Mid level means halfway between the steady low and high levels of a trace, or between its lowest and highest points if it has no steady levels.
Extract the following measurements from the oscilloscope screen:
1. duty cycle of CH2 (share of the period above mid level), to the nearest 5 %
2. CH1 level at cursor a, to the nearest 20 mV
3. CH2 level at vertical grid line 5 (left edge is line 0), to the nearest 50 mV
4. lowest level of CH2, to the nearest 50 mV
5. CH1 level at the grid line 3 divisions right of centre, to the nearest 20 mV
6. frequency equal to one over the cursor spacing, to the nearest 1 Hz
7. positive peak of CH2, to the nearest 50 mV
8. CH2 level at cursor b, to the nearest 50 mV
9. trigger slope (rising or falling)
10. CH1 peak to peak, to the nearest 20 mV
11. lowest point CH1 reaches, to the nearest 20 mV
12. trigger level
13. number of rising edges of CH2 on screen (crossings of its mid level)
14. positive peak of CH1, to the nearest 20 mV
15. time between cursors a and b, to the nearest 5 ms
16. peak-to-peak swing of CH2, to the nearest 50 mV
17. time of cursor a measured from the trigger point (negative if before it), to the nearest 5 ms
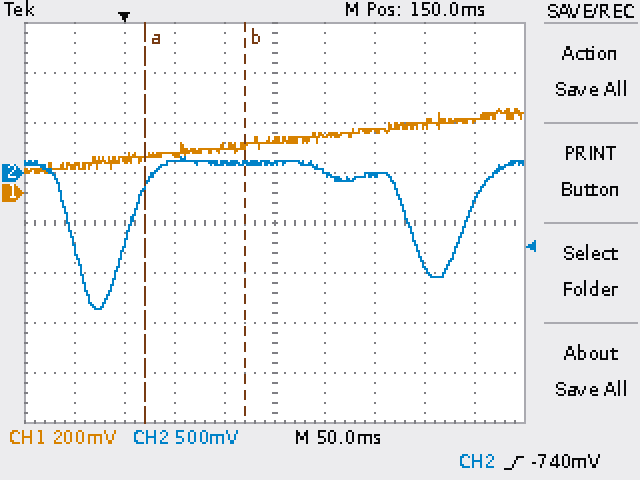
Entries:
85 %
140 mV
100 mV
-1.35 V
280 mV
10 Hz
150 mV
100 mV
rising
260 mV
80 mV
-740 mV
2
340 mV
100 ms
1.50 V
+20 ms
